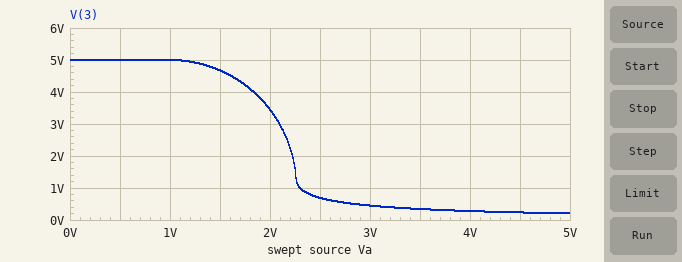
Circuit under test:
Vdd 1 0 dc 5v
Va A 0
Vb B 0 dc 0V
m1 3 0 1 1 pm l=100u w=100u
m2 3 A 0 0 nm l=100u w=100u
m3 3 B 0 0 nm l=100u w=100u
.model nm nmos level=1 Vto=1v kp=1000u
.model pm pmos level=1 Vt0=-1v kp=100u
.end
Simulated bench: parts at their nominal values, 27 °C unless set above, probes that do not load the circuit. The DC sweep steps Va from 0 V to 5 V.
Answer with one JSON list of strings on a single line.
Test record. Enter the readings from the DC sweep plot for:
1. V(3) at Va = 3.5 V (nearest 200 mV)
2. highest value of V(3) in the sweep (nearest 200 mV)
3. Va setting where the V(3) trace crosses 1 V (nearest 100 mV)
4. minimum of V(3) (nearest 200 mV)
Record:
["400 mV", "5.0 V", "2.3 V", "200 mV"]
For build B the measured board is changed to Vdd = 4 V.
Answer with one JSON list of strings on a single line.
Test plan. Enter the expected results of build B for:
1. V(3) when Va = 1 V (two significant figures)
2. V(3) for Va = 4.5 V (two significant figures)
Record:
["4.0 V", "130 mV"]
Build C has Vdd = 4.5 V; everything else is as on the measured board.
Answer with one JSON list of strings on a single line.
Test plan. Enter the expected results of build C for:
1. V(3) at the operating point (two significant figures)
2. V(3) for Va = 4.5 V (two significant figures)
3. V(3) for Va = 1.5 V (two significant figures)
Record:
["4.5 V", "180 mV", "4.1 V"]
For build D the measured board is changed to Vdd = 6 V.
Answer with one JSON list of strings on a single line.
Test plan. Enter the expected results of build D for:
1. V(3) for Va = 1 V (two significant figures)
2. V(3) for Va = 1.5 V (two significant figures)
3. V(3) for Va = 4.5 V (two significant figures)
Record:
["6.0 V", "5.7 V", "380 mV"]
